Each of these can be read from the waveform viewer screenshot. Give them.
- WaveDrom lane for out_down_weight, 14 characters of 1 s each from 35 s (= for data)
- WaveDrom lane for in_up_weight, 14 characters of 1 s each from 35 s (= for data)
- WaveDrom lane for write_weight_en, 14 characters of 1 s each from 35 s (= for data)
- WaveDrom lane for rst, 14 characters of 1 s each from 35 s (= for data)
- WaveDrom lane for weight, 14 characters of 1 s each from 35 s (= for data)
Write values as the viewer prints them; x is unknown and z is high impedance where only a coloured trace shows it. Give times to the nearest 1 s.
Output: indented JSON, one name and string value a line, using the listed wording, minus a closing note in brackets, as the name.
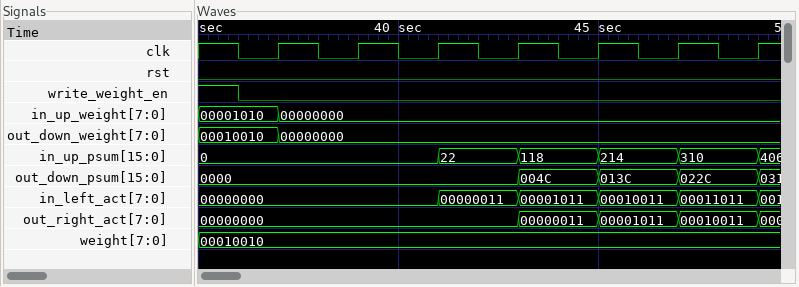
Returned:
{
  "WaveDrom lane for out_down_weight, 14 characters of 1 s each from 35 s": "{name: 'out_down_weight', wave: '=.=...........', data: '00010010 00000000'}",
  "WaveDrom lane for in_up_weight, 14 characters of 1 s each from 35 s": "{name: 'in_up_weight', wave: '=.=...........', data: '00001010 00000000'}",
  "WaveDrom lane for write_weight_en, 14 characters of 1 s each from 35 s": "{name: 'write_weight_en', wave: '10............'}",
  "WaveDrom lane for rst, 14 characters of 1 s each from 35 s": "{name: 'rst', wave: '0.............'}",
  "WaveDrom lane for weight, 14 characters of 1 s each from 35 s": "{name: 'weight', wave: '=.............', data: '00010010'}"
}
